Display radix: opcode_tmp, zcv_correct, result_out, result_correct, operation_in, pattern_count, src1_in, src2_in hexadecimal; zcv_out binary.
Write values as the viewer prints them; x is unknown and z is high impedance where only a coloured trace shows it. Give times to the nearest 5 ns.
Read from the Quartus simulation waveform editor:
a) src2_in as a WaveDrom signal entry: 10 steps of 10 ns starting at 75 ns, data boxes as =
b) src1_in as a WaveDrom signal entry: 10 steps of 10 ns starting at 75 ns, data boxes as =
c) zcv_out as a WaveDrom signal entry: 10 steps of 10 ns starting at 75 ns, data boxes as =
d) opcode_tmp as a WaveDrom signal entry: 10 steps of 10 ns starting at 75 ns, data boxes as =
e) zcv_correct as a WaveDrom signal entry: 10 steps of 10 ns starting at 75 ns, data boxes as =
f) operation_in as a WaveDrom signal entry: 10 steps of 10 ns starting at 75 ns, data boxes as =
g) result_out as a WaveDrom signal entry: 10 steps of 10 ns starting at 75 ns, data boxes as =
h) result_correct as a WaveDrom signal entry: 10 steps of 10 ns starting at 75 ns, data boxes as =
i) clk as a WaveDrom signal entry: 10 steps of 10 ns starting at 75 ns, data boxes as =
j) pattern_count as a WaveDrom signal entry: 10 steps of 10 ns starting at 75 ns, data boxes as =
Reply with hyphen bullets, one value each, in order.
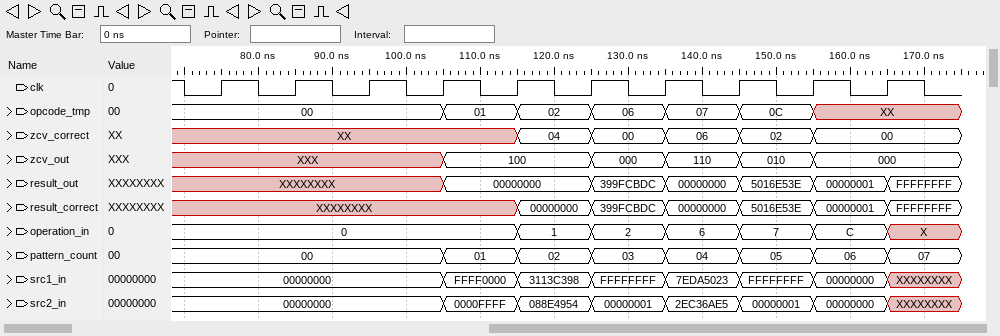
- {name: 'src2_in', wave: '=..======x', data: '00000000 0000FFFF 088E4954 00000001 2EC36AE5 00000001 00000000'}
- {name: 'src1_in', wave: '=..======x', data: '00000000 FFFF0000 3113C398 FFFFFFFF 7EDA5023 FFFFFFFF 00000000'}
- {name: 'zcv_out', wave: 'x..=.====.', data: '100 000 110 010 000'}
- {name: 'opcode_tmp', wave: '=..=====x.', data: '00 01 02 06 07 0C'}
- {name: 'zcv_correct', wave: 'x...=====.', data: '04 00 06 02 00'}
- {name: 'operation_in', wave: '=...=====x', data: '0 1 2 6 7 C'}
- {name: 'result_out', wave: 'x..=.=====', data: '00000000 399FCBDC 00000000 5016E53E 00000001 FFFFFFFF'}
- {name: 'result_correct', wave: 'x...======', data: '00000000 399FCBDC 00000000 5016E53E 00000001 FFFFFFFF'}
- {name: 'clk', wave: 'p.........'}
- {name: 'pattern_count', wave: '=..=======', data: '00 01 02 03 04 05 06 07'}
